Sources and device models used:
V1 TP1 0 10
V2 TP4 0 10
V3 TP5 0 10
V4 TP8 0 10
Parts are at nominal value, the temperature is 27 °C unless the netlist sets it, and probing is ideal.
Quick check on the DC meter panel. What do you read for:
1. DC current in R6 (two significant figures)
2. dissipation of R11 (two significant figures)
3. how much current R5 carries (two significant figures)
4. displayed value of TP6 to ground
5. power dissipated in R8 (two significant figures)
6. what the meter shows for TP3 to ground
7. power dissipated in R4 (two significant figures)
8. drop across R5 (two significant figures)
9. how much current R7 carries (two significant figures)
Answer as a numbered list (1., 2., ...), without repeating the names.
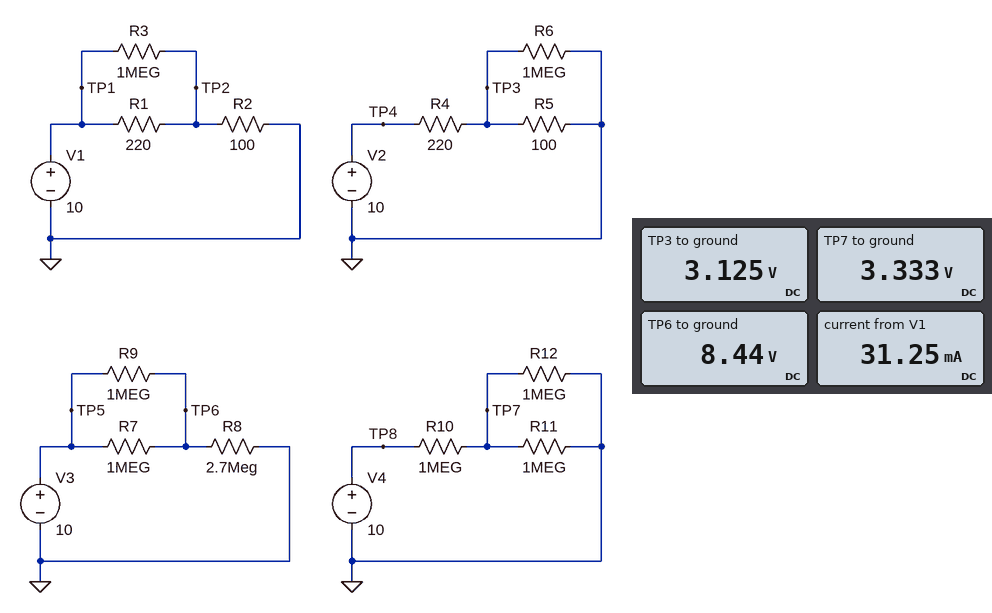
1. 3.1 µA
2. 11 µW
3. 31 mA
4. 8.44 V
5. 26 µW
6. 3.125 V
7. 210 mW
8. 3.1 V
9. 1.6 µA
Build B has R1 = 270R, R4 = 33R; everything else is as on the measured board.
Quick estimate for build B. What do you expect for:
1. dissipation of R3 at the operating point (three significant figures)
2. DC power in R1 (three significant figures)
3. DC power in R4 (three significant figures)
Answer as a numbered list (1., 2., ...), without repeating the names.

1. 53.2 µW
2. 197 mW
3. 187 mW
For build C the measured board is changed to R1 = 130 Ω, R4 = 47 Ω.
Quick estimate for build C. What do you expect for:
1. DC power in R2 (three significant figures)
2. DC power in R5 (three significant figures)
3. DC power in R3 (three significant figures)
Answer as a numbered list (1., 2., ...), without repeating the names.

1. 189 mW
2. 463 mW
3. 31.9 µW
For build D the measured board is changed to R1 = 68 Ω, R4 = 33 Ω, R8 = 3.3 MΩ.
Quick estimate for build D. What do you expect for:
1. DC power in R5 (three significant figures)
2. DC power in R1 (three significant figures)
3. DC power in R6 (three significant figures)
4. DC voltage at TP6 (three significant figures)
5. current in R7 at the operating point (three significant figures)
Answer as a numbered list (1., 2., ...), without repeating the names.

1. 565 mW
2. 241 mW
3. 56.5 µW
4. 8.68 V
5. 1.32 µA
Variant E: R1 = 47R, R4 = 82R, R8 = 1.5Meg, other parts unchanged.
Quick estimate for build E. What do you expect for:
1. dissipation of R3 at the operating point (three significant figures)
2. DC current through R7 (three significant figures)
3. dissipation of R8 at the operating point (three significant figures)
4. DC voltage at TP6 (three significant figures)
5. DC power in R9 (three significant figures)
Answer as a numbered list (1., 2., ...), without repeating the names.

1. 10.2 µW
2. 2.50 µA
3. 37.5 µW
4. 7.50 V
5. 6.25 µW
